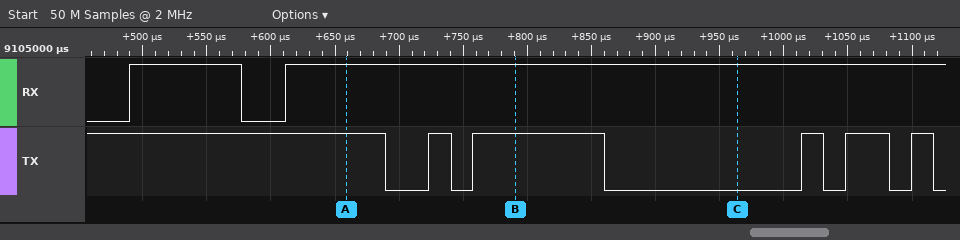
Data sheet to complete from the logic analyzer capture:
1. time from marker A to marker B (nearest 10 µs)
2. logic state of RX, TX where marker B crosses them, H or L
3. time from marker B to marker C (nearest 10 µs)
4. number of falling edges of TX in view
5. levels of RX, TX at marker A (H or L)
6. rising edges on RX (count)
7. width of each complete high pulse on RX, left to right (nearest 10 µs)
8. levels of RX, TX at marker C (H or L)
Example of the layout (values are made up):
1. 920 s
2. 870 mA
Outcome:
1. 130 µs
2. RX=H, TX=H
3. 170 µs
4. 6
5. RX=H, TX=H
6. 2
7. 90 µs
8. RX=H, TX=L
